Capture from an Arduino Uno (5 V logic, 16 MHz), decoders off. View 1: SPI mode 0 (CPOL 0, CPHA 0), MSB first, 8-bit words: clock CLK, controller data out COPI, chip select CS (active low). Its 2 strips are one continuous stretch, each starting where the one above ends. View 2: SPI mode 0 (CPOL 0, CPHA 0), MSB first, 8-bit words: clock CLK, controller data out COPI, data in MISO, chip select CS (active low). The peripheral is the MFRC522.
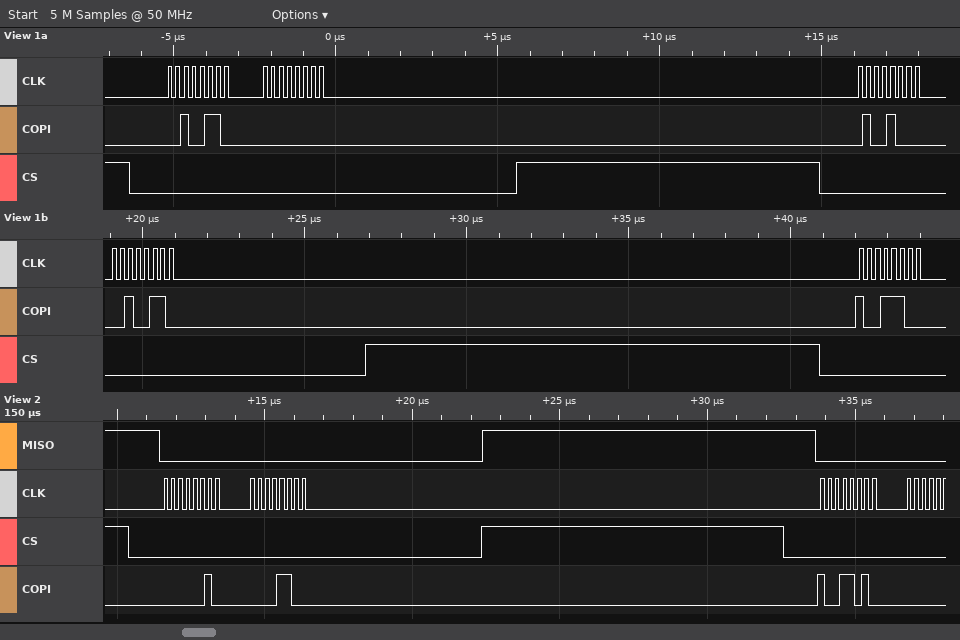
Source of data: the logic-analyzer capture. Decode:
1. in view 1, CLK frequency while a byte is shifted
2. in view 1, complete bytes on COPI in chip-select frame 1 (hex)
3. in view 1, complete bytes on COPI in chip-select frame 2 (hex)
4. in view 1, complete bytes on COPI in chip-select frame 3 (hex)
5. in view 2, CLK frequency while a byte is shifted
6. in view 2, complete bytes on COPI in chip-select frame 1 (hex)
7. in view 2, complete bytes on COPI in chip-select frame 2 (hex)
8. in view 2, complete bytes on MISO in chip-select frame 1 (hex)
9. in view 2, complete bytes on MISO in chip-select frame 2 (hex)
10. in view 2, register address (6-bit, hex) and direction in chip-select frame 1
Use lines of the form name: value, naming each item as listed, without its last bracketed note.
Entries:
in view 1, CLK frequency while a byte is shifted: 4 MHz
in view 1, complete bytes on COPI in chip-select frame 1: 26 00
in view 1, complete bytes on COPI in chip-select frame 2: 48 26
in view 1, complete bytes on COPI in chip-select frame 3: 9C
in view 2, CLK frequency while a byte is shifted: 4 MHz
in view 2, complete bytes on COPI in chip-select frame 1: 02 0C
in view 2, complete bytes on COPI in chip-select frame 2: 9A
in view 2, complete bytes on MISO in chip-select frame 1: 00 00
in view 2, complete bytes on MISO in chip-select frame 2: 00
in view 2, register address (6-bit, hex) and direction in chip-select frame 1: 0x01 write
